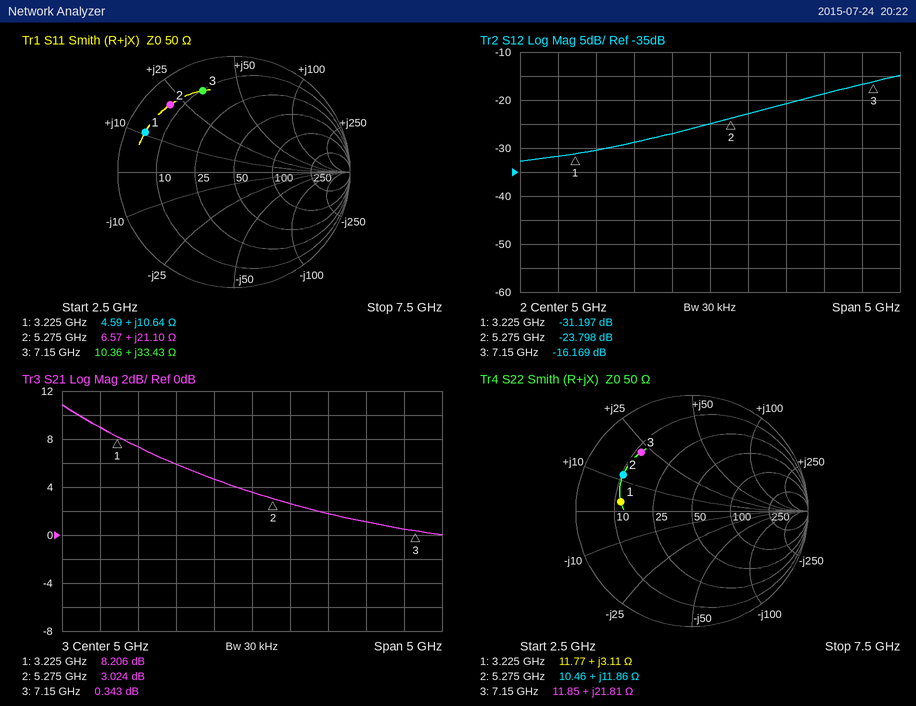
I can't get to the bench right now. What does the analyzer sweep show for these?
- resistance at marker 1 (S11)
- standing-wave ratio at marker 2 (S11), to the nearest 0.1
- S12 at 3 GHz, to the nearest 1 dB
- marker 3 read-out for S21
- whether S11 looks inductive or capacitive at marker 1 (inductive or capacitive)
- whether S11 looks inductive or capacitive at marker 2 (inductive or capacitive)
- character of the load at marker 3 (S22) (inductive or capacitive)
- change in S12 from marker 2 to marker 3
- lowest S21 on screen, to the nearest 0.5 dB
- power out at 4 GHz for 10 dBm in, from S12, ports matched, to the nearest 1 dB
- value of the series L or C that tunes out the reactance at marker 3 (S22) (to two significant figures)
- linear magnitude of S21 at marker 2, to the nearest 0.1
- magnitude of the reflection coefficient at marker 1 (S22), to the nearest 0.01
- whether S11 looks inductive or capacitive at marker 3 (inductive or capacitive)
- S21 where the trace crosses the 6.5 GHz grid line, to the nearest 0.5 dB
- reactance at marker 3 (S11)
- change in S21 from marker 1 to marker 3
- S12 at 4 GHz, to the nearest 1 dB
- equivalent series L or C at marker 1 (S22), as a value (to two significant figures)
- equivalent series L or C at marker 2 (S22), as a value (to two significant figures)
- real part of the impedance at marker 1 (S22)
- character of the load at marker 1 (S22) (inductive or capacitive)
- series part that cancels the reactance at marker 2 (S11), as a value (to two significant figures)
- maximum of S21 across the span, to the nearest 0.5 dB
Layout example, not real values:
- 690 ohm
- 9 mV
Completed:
- 4.59 Ω
- 9.0
- -32 dB
- 0.343 dB
- inductive
- inductive
- inductive
- 7.629 dB
- 0.0 dB
- -19 dBm
- 1.0 pF
- 1.4
- 0.62
- inductive
- 1.0 dB
- +33.43 Ω
- -7.863 dB
- -29 dB
- 150 pH
- 360 pH
- 11.77 Ω
- inductive
- 1.4 pF
- 11.0 dB
